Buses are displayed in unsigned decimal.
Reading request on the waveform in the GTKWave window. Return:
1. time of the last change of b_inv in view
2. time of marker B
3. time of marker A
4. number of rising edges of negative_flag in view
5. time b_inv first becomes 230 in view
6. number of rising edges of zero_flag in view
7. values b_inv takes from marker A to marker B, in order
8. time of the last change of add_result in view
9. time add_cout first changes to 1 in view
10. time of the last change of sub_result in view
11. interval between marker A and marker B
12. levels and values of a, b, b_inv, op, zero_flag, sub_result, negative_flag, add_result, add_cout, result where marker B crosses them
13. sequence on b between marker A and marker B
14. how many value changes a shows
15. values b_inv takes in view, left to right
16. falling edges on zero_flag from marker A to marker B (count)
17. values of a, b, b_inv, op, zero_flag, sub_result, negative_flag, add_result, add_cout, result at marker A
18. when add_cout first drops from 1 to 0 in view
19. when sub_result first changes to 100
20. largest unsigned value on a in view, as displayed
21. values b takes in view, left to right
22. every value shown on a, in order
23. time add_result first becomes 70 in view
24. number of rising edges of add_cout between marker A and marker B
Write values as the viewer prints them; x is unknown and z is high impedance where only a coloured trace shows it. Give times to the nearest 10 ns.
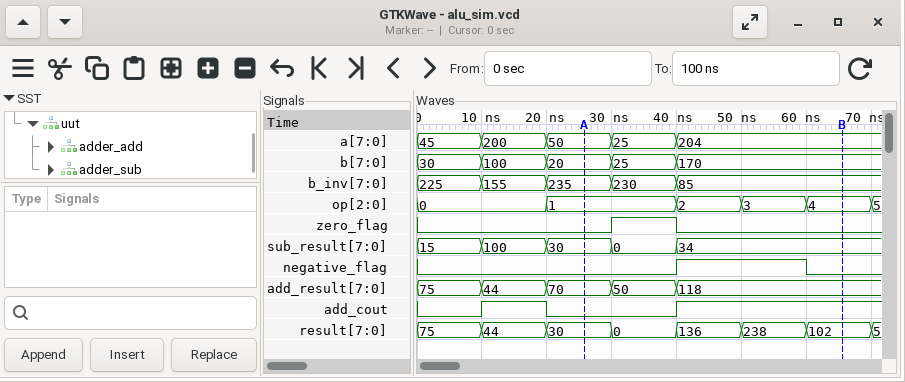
40 ns
70 ns
30 ns
1
30 ns
1
235, 230, 85
40 ns
10 ns
40 ns
40 ns
a=204, b=170, b_inv=85, op=4, zero_flag=0, sub_result=34, negative_flag=0, add_result=118, add_cout=1, result=102
20, 25, 170
4
225, 155, 235, 230, 85
1
a=50, b=20, b_inv=235, op=1, zero_flag=0, sub_result=30, negative_flag=0, add_result=70, add_cout=0, result=30
20 ns
10 ns
204
30, 100, 20, 25, 170
45, 200, 50, 25, 204
20 ns
1
